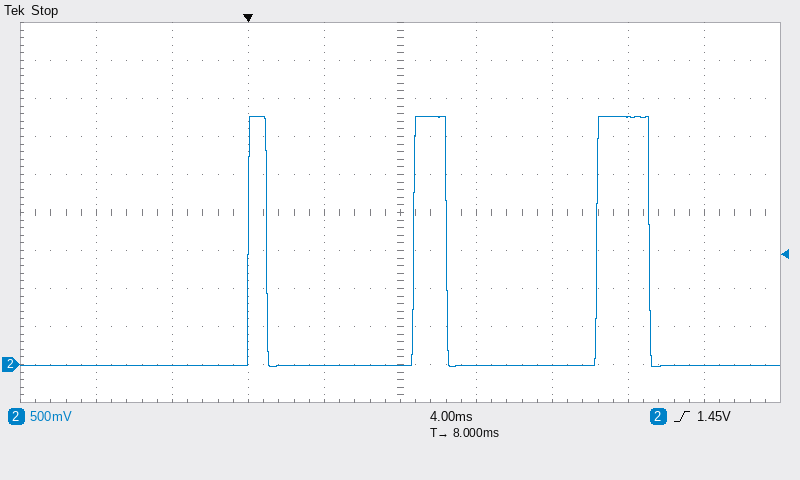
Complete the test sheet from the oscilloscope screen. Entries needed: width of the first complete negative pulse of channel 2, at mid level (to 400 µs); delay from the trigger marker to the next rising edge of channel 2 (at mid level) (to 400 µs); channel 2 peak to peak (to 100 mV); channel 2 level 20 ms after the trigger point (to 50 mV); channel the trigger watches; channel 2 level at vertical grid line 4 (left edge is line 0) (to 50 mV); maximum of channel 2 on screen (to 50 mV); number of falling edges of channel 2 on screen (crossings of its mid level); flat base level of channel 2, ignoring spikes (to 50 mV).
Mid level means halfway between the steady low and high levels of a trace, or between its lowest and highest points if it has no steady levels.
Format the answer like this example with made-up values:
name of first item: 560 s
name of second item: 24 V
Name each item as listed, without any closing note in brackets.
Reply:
width of the first complete negative pulse of channel 2, at mid level: 7.6 ms
delay from the trigger marker to the next rising edge of channel 2 (at mid level): 8.8 ms
channel 2 peak to peak: 3.30 V
channel 2 level 20 ms after the trigger point: 3.25 V
channel the trigger watches: channel 2
channel 2 level at vertical grid line 4 (left edge is line 0): 0 mV
maximum of channel 2 on screen: 3.25 V
number of falling edges of channel 2 on screen: 3
flat base level of channel 2, ignoring spikes: 0 mV
